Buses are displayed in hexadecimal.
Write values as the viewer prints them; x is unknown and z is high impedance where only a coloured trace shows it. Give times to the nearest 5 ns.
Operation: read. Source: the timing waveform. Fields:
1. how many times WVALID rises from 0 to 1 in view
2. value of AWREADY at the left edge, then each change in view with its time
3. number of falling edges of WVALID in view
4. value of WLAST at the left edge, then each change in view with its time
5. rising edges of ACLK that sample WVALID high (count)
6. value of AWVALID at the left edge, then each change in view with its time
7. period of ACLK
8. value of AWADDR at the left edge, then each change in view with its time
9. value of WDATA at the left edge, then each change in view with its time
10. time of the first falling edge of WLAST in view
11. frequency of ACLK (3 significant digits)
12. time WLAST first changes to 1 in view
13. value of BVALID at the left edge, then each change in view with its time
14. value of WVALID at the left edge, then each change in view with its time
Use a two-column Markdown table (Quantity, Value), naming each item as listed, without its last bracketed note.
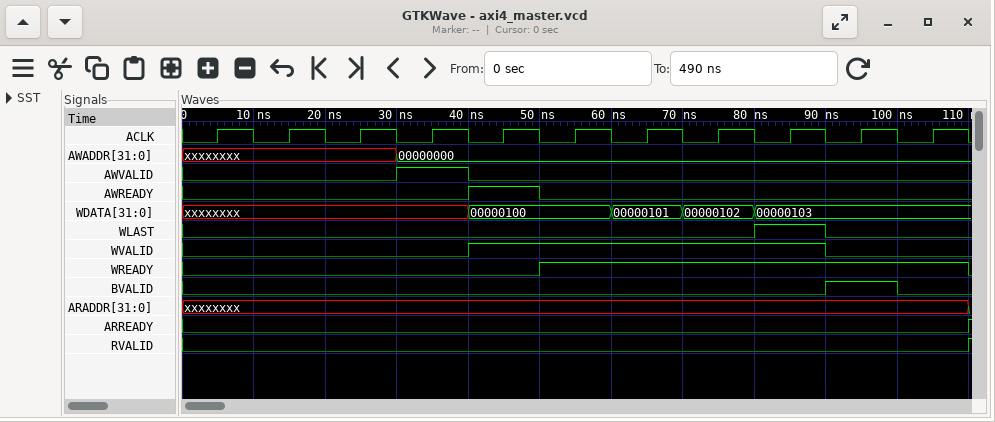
| Quantity | Value |
|---|---|
| how many times WVALID rises from 0 to 1 in view | 1 |
| value of AWREADY at the left edge, then each change in view with its time | 0, 1 at 40 ns, 0 at 50 ns |
| number of falling edges of WVALID in view | 1 |
| value of WLAST at the left edge, then each change in view with its time | 0, 1 at 80 ns, 0 at 90 ns |
| rising edges of ACLK that sample WVALID high | 5 |
| value of AWVALID at the left edge, then each change in view with its time | 0, 1 at 30 ns, 0 at 40 ns |
| period of ACLK | 10 ns |
| value of AWADDR at the left edge, then each change in view with its time | xxxxxxxx, 00000000 at 30 ns |
| value of WDATA at the left edge, then each change in view with its time | xxxxxxxx, 00000100 at 40 ns, 00000101 at 60 ns, 00000102 at 70 ns, 00000103 at 80 ns |
| time of the first falling edge of WLAST in view | 90 ns |
| frequency of ACLK | 100 MHz |
| time WLAST first changes to 1 in view | 80 ns |
| value of BVALID at the left edge, then each change in view with its time | 0, 1 at 90 ns, 0 at 100 ns |
| value of WVALID at the left edge, then each change in view with its time | 0, 1 at 40 ns, 0 at 90 ns |
